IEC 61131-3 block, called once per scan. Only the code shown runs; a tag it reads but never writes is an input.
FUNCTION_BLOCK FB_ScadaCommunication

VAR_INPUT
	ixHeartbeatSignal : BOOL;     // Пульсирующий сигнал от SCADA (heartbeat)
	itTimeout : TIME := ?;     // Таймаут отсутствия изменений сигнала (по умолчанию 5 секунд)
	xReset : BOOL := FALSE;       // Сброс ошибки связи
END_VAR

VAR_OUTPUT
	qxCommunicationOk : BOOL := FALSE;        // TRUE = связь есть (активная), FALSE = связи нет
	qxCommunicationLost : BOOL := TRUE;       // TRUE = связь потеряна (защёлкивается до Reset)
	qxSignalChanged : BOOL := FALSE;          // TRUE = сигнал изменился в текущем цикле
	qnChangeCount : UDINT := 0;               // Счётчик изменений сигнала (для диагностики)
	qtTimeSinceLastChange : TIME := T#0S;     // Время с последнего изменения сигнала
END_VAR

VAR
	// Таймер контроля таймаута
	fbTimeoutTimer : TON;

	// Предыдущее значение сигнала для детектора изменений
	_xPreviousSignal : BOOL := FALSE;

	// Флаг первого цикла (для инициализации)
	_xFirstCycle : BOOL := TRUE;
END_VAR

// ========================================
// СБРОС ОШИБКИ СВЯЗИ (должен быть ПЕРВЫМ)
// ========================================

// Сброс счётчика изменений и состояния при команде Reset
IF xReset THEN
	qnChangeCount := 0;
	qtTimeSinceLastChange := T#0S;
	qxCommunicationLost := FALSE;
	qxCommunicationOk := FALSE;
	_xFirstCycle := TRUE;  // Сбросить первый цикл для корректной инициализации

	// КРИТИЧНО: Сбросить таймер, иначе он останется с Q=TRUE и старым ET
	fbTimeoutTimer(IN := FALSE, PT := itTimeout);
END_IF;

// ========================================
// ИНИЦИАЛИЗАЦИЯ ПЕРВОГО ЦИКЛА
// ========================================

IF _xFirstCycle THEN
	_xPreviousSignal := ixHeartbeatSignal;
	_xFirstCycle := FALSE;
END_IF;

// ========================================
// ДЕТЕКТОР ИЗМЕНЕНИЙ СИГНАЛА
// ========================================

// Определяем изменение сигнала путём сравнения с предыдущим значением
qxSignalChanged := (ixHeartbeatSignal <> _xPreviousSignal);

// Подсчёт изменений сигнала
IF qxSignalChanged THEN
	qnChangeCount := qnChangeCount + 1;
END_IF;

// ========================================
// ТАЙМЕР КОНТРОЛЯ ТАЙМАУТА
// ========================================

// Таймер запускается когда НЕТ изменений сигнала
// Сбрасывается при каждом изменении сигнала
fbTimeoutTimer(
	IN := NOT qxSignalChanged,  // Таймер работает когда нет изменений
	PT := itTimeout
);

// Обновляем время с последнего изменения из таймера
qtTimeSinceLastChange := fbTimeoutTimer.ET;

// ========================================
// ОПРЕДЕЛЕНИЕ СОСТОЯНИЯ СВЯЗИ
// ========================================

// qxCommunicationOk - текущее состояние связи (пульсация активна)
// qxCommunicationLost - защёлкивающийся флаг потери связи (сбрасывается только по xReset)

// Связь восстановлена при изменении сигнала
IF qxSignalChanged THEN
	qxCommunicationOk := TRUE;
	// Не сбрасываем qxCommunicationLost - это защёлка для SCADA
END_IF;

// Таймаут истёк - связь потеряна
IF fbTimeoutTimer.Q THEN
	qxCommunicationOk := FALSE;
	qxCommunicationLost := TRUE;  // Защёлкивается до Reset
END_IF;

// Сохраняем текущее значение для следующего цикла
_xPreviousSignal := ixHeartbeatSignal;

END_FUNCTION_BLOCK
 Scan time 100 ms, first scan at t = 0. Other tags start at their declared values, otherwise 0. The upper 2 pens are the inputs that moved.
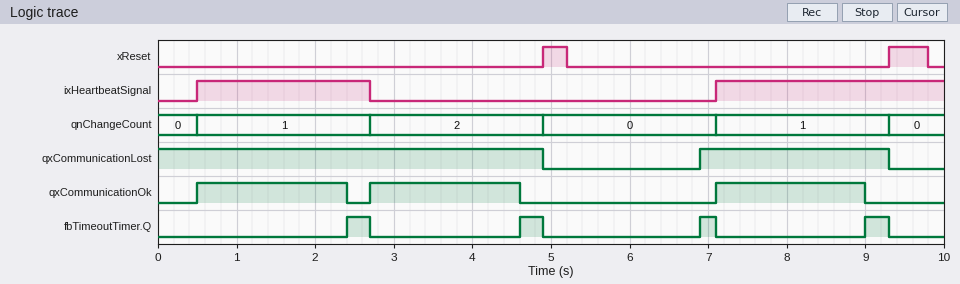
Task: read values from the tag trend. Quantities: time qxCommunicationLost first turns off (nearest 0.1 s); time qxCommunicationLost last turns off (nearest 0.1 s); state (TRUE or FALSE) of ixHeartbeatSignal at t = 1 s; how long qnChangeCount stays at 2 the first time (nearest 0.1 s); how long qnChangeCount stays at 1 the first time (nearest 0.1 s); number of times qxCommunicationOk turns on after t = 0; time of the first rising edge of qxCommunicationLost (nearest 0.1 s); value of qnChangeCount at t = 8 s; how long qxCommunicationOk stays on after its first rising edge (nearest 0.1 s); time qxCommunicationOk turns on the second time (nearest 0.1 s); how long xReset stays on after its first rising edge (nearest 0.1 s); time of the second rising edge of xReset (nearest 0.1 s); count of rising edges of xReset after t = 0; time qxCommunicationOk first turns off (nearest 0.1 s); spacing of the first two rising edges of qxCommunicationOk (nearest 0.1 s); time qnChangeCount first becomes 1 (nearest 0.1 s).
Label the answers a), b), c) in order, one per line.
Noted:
a) 4.9 s
b) 9.3 s
c) TRUE
d) 2.2 s
e) 2.2 s
f) 3
g) 6.9 s
h) 1
i) 1.9 s
j) 2.7 s
k) 0.3 s
l) 9.3 s
m) 2
n) 2.4 s
o) 2.2 s
p) 0.5 s
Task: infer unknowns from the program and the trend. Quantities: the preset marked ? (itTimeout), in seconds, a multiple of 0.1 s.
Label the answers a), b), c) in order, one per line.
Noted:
a) 1.8 s
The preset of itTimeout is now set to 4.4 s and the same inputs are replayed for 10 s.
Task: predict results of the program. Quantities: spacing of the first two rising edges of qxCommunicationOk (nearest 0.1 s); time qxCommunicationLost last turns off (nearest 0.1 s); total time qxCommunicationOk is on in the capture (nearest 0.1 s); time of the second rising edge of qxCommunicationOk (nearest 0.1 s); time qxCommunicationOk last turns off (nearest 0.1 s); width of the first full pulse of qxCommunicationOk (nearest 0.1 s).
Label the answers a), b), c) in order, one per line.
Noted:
a) 6.6 s
b) 4.9 s
c) 6.6 s
d) 7.1 s
e) 9.3 s
f) 4.4 s
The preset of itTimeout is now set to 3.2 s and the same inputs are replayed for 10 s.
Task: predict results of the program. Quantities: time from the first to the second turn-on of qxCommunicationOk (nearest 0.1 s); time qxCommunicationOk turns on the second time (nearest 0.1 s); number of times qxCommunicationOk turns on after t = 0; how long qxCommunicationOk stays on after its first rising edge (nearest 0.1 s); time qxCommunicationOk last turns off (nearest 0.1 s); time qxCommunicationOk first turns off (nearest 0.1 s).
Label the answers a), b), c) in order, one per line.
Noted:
a) 6.6 s
b) 7.1 s
c) 2
d) 4.4 s
e) 9.3 s
f) 4.9 s
